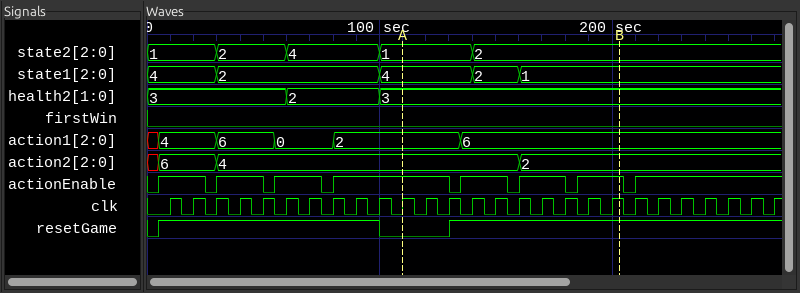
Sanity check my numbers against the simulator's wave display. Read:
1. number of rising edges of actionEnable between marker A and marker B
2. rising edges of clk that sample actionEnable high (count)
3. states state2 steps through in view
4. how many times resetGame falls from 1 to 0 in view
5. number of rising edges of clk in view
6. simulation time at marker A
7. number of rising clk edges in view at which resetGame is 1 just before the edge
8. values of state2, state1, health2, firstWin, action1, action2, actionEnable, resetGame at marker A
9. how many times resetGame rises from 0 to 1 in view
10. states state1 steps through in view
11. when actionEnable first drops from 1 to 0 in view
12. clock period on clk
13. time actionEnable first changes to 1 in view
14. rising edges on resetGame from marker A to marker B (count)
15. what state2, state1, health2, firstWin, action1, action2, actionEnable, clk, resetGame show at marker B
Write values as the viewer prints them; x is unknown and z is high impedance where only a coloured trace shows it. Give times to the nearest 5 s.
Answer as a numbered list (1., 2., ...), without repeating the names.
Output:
1. 3
2. 23
3. 1, 2, 4, 1, 2
4. 1
5. 27
6. 110 s
7. 24
8. state2=1, state1=4, health2=3, firstWin=0, action1=2, action2=4, actionEnable=1, resetGame=0
9. 2
10. 4, 2, 4, 2, 1
11. 25 s
12. 10 s
13. 5 s
14. 1
15. state2=2, state1=1, health2=3, firstWin=0, action1=6, action2=2, actionEnable=1, clk=1, resetGame=1
